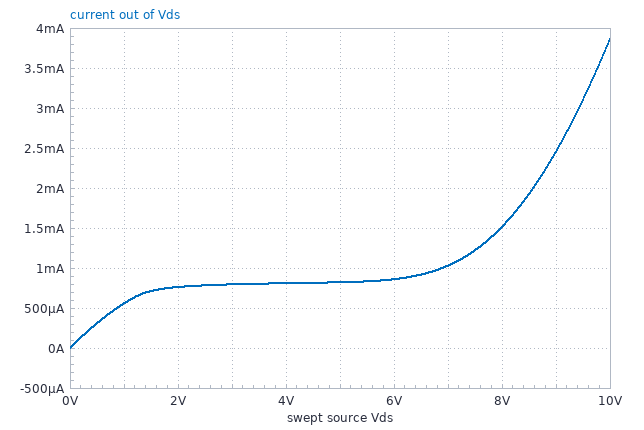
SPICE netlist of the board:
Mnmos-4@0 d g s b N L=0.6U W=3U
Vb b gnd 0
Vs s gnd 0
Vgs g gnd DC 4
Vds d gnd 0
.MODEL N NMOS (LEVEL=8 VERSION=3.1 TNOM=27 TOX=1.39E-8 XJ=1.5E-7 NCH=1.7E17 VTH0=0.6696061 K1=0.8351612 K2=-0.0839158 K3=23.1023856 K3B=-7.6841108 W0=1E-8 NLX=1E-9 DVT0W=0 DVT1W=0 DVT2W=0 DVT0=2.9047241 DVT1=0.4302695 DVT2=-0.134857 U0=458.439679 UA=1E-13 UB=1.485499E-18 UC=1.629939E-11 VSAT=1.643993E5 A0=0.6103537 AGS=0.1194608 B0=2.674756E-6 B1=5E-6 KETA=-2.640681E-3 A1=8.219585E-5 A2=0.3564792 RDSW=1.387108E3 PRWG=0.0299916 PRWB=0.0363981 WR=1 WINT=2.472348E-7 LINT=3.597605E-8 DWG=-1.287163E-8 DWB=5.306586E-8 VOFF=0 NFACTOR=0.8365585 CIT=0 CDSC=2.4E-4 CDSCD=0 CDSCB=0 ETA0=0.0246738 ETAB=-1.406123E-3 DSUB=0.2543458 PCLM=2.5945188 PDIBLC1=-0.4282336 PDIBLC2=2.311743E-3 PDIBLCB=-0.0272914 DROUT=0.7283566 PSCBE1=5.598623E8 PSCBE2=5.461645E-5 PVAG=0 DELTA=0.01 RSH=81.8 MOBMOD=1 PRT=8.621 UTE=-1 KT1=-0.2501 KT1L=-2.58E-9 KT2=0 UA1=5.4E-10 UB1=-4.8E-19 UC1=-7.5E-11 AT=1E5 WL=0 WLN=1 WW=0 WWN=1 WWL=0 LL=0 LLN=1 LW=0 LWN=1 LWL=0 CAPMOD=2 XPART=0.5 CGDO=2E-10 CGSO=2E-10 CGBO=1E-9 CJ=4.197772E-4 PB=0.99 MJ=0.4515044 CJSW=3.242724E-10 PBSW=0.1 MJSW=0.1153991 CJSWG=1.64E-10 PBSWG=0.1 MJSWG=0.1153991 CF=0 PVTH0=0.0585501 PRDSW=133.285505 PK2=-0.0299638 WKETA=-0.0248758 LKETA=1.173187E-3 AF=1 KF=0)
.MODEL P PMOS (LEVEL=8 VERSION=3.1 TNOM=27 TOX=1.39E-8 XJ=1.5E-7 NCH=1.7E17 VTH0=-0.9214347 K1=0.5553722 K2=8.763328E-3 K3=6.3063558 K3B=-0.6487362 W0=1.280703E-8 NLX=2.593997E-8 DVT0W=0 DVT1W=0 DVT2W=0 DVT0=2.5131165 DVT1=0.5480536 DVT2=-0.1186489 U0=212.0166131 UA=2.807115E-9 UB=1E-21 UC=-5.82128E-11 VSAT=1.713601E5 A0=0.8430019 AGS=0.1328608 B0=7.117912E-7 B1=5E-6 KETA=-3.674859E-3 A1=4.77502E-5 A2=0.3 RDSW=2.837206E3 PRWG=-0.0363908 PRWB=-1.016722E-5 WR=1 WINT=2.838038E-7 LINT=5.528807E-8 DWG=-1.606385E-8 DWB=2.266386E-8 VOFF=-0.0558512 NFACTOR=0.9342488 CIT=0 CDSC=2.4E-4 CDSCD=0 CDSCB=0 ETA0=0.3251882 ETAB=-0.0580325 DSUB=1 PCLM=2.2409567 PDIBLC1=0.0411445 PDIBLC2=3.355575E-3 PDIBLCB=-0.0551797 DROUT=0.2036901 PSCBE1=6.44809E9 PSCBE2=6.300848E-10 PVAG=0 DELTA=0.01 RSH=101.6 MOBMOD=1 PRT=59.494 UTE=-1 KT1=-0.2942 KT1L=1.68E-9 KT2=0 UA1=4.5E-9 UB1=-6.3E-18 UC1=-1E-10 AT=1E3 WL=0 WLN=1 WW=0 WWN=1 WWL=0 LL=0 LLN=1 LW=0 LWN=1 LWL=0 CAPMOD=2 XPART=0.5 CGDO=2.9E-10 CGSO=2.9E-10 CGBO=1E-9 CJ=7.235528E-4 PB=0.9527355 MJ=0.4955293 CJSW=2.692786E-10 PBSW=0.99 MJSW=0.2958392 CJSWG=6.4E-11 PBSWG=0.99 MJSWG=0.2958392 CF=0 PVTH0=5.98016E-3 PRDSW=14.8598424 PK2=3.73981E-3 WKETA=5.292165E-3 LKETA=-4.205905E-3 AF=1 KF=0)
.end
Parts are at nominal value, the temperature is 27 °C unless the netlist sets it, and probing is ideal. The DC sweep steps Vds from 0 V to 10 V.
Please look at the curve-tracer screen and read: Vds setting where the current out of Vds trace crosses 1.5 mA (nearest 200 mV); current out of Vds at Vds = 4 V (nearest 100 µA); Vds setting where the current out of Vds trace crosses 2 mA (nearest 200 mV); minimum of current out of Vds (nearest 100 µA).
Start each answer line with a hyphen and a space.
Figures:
- 8.0 V
- 800 µA
- 8.6 V
- 0 A
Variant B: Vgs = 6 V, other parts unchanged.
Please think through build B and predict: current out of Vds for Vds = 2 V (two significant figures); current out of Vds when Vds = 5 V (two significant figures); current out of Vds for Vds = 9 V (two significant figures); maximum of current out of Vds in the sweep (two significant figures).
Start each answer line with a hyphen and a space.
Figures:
- 1.2 mA
- 1.4 mA
- 2.9 mA
- 4.5 mA
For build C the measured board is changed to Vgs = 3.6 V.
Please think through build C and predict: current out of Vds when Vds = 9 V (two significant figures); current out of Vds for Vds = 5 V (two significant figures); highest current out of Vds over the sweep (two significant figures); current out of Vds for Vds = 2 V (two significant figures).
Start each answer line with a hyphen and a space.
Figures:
- 2.3 mA
- 710 µA
- 3.6 mA
- 660 µA
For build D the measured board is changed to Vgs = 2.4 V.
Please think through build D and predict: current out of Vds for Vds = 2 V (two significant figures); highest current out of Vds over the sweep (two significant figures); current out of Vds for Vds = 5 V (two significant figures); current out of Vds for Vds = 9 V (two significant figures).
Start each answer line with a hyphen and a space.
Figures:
- 340 µA
- 2.4 mA
- 370 µA
- 1.5 mA
